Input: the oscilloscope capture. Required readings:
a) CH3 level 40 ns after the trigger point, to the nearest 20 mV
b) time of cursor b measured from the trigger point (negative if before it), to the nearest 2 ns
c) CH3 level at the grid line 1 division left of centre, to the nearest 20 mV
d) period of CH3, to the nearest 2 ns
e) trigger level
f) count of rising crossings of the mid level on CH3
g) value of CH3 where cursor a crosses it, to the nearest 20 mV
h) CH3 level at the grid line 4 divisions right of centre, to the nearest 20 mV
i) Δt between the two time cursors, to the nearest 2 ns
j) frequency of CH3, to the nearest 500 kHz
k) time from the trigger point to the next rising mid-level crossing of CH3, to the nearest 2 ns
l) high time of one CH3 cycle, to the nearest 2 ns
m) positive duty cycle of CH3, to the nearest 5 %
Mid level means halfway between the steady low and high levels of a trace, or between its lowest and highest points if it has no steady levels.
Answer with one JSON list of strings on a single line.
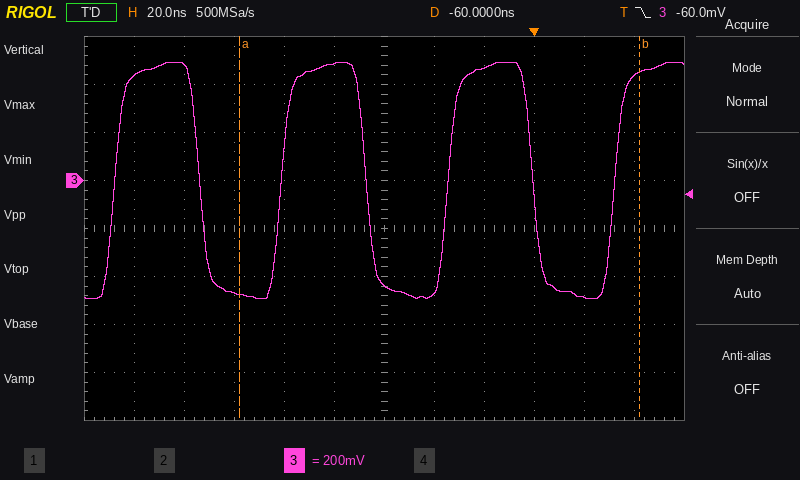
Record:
["440 mV", "+42 ns", "480 mV", "66 ns", "-60.0 mV", "4", "-480 mV", "-480 mV", "160 ns", "15.0 MHz", "32 ns", "34 ns", "50 %"]
